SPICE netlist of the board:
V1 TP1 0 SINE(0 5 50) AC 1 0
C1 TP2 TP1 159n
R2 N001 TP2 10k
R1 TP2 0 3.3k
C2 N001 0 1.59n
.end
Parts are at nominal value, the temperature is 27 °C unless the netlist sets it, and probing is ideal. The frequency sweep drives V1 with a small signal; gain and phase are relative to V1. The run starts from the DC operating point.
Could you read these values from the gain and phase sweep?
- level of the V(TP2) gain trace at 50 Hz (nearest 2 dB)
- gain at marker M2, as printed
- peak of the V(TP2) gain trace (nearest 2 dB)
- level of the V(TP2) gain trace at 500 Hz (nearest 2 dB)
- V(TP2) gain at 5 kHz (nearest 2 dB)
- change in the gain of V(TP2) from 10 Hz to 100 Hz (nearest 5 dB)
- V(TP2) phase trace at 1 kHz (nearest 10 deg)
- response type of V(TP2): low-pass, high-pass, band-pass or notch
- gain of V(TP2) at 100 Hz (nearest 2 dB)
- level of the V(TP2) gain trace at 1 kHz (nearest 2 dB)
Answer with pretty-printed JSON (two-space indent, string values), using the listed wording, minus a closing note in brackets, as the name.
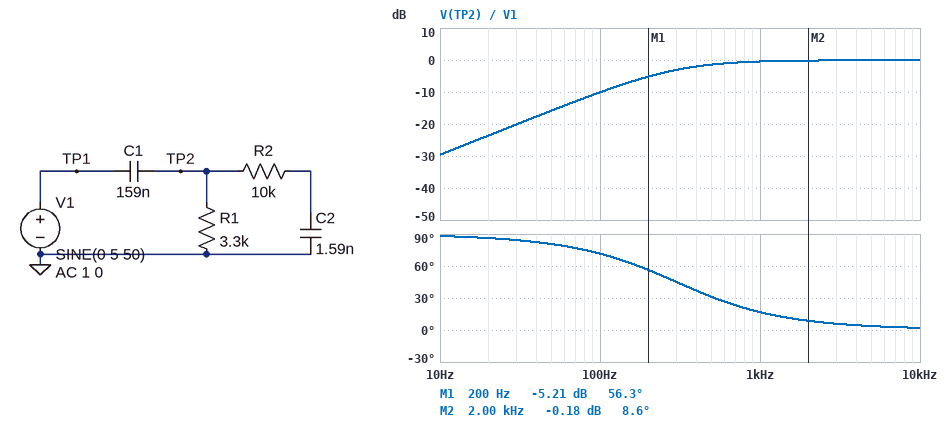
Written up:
{
  "level of the V(TP2) gain trace at 50 Hz": "-16 dB",
  "gain at marker M2, as printed": "-0.18 dB",
  "peak of the V(TP2) gain trace": "0 dB",
  "level of the V(TP2) gain trace at 500 Hz": "-2 dB",
  "V(TP2) gain at 5 kHz": "0 dB",
  "change in the gain of V(TP2) from 10 Hz to 100 Hz": "20 dB",
  "V(TP2) phase trace at 1 kHz": "20 deg",
  "response type of V(TP2): low-pass, high-pass, band-pass or notch": "high-pass",
  "gain of V(TP2) at 100 Hz": "-10 dB",
  "level of the V(TP2) gain trace at 1 kHz": "0 dB"
}
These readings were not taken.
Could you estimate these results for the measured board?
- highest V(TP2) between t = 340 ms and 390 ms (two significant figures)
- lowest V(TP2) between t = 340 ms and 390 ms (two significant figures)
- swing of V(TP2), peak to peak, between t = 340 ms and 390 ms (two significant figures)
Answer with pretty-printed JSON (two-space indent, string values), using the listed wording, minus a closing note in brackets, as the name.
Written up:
{
  "highest V(TP2) between t = 340 ms and 390 ms": "810 mV",
  "lowest V(TP2) between t = 340 ms and 390 ms": "-810 mV",
  "swing of V(TP2), peak to peak, between t = 340 ms and 390 ms": "1.6 V"
}
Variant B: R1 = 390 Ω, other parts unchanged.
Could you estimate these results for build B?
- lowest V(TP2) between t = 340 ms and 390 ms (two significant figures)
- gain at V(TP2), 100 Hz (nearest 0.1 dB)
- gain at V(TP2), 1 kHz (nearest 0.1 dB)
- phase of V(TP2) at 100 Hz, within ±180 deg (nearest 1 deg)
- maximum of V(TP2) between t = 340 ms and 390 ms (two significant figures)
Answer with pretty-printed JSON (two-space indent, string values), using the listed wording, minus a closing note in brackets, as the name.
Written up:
{
  "lowest V(TP2) between t = 340 ms and 390 ms": "-97 mV",
  "gain at V(TP2), 100 Hz": "-28.2 dB",
  "gain at V(TP2), 1 kHz": "-8.8 dB",
  "phase of V(TP2) at 100 Hz, within ±180 deg": "88 deg",
  "maximum of V(TP2) between t = 340 ms and 390 ms": "97 mV"
}
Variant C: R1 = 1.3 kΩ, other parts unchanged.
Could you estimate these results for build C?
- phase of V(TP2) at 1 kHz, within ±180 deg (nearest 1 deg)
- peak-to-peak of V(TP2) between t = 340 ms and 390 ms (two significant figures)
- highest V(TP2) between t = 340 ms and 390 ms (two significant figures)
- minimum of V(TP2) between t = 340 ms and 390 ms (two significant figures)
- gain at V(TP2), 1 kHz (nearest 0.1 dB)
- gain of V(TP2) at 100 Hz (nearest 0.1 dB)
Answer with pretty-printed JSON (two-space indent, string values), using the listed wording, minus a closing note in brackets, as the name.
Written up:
{
  "phase of V(TP2) at 1 kHz, within ±180 deg": "37 deg",
  "peak-to-peak of V(TP2) between t = 340 ms and 390 ms": "650 mV",
  "highest V(TP2) between t = 340 ms and 390 ms": "320 mV",
  "minimum of V(TP2) between t = 340 ms and 390 ms": "-320 mV",
  "gain at V(TP2), 1 kHz": "-2.1 dB",
  "gain of V(TP2) at 100 Hz": "-17.8 dB"
}
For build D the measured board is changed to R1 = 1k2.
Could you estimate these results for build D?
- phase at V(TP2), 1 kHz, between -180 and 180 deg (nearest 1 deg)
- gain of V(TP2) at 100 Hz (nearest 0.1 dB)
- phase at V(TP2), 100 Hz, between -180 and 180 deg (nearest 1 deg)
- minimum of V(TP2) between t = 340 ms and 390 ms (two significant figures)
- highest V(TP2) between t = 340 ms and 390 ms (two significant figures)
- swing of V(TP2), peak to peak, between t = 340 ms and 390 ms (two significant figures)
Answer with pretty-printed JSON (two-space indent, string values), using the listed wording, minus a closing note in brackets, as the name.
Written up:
{
  "phase at V(TP2), 1 kHz, between -180 and 180 deg": "40 deg",
  "gain of V(TP2) at 100 Hz": "-18.5 dB",
  "phase at V(TP2), 100 Hz, between -180 and 180 deg": "83 deg",
  "minimum of V(TP2) between t = 340 ms and 390 ms": "-300 mV",
  "highest V(TP2) between t = 340 ms and 390 ms": "300 mV",
  "swing of V(TP2), peak to peak, between t = 340 ms and 390 ms": "600 mV"
}
